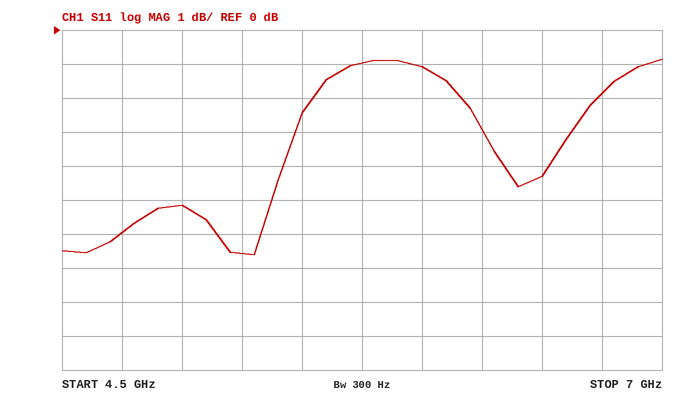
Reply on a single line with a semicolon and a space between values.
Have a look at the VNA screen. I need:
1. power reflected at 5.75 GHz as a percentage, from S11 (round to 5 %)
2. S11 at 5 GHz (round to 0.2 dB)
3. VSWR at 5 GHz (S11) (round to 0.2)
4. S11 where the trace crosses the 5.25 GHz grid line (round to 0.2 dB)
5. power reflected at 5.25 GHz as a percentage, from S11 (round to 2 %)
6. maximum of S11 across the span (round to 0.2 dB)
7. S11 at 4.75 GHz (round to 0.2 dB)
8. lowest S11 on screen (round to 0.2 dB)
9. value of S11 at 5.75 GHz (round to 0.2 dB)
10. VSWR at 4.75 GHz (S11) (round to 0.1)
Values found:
80 %; -5.2 dB; 3.4; -6.6 dB; 22 %; -0.8 dB; -6.0 dB; -6.6 dB; -1.0 dB; 3.0
